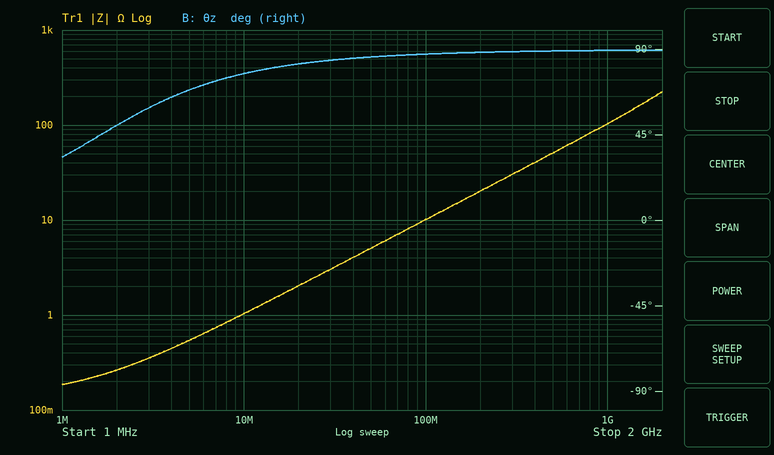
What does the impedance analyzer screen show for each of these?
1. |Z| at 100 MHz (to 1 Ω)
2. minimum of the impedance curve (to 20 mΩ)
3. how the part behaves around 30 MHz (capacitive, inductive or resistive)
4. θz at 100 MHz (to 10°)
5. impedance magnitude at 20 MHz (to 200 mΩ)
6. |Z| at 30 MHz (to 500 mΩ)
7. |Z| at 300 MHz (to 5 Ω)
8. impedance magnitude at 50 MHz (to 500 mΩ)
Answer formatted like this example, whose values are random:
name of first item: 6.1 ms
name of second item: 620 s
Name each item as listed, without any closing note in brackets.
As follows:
|Z| at 100 MHz: 10 Ω
minimum of the impedance curve: 180 mΩ
how the part behaves around 30 MHz: inductive
θz at 100 MHz: 90°
impedance magnitude at 20 MHz: 2.0 Ω
|Z| at 30 MHz: 3.0 Ω
|Z| at 300 MHz: 30 Ω
impedance magnitude at 50 MHz: 5.0 Ω
